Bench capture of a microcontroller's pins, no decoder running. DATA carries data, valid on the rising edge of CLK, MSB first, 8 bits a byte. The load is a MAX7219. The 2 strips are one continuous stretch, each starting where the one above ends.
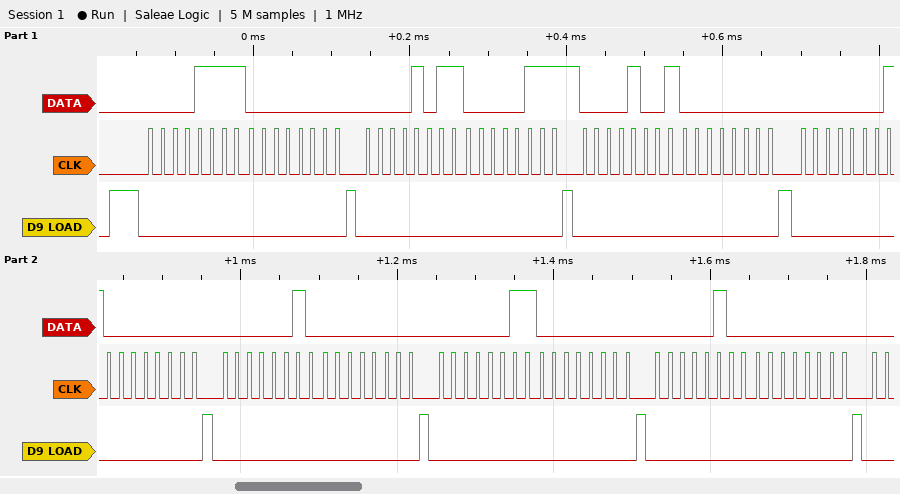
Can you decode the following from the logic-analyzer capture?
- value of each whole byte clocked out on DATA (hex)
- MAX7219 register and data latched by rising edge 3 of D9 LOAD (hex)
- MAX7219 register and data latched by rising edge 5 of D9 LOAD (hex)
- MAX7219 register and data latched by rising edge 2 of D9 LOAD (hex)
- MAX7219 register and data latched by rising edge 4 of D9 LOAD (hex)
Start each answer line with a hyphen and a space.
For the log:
- 0F 00 0B 07 09 00 01 00 02 00 03 00 04 00
- register 0xB, data 0x07
- register 0x1, data 0x00
- register 0xF, data 0x00
- register 0x9, data 0x00
